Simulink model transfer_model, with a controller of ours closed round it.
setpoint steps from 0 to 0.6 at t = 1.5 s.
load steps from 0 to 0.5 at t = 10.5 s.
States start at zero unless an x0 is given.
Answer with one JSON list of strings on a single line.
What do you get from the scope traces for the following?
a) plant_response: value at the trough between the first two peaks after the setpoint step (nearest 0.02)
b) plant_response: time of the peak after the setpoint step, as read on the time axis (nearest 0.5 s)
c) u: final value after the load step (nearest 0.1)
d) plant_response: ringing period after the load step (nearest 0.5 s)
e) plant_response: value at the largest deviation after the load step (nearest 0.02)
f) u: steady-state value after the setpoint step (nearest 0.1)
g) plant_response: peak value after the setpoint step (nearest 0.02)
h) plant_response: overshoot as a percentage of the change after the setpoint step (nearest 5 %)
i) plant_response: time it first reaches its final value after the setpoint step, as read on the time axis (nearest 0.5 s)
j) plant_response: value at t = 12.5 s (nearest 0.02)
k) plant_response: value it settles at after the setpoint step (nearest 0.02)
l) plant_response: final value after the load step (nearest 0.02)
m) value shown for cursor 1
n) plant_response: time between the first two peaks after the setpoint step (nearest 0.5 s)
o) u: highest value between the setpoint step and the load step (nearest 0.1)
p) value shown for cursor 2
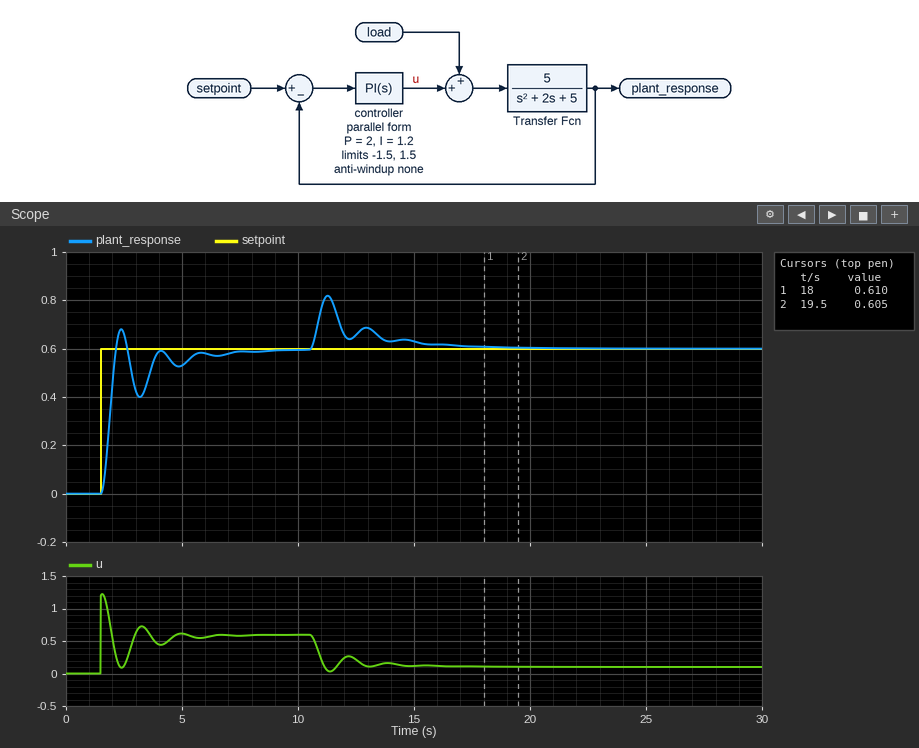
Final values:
["0.40", "2.5 s", "0.1", "1.5 s", "0.82", "0.6", "0.68", "15 %", "2.0 s", "0.66", "0.60", "0.60", "0.610", "1.5 s", "1.2", "0.605"]
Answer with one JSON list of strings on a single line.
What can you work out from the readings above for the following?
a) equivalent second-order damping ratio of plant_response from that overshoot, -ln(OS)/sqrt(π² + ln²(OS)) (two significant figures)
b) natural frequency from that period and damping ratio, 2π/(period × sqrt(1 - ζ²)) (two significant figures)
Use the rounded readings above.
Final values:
["0.52", "4.9 rad/s"]
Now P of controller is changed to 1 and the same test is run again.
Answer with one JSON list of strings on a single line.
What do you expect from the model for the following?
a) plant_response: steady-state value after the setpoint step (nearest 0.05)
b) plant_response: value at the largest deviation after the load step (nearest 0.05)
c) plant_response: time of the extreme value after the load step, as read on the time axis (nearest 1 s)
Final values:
["0.60", "0.90", "11 s"]
